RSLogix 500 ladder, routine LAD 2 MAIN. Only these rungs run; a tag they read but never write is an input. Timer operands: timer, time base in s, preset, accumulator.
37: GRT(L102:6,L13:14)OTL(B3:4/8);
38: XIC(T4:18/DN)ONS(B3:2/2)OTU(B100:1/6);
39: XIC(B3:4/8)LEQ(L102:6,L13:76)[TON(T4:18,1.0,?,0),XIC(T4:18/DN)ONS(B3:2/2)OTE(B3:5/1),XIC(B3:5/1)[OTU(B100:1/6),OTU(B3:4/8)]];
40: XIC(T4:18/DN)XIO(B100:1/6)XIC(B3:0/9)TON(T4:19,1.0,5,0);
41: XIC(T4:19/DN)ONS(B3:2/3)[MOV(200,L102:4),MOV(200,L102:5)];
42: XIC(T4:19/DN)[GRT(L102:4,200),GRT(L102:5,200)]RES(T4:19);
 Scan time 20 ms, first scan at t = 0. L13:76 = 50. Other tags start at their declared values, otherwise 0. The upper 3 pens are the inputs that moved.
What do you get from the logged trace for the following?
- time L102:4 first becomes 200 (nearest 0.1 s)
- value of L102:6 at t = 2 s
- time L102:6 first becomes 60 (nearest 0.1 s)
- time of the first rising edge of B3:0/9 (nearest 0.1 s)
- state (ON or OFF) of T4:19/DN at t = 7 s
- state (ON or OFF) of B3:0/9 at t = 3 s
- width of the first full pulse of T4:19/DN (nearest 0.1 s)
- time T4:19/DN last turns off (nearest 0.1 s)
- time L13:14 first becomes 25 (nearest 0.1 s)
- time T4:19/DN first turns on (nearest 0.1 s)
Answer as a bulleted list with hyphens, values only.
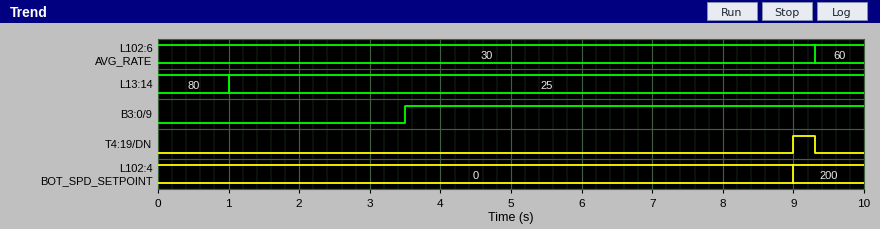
- 9.0 s
- 30
- 9.3 s
- 3.5 s
- OFF
- OFF
- 0.3 s
- 9.3 s
- 1.0 s
- 9.0 s
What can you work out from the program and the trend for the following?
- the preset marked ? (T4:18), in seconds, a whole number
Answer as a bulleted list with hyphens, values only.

- 3 s
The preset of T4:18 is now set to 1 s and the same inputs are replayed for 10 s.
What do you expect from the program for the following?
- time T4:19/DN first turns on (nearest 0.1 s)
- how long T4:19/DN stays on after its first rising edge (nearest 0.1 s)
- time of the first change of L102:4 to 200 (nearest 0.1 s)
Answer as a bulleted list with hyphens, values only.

- 8.5 s
- 0.8 s
- 8.5 s
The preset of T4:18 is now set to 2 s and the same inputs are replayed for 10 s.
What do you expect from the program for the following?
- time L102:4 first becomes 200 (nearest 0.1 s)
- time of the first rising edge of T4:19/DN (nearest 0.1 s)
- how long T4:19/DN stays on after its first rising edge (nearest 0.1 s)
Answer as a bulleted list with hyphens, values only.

- 8.5 s
- 8.5 s
- 0.8 s
